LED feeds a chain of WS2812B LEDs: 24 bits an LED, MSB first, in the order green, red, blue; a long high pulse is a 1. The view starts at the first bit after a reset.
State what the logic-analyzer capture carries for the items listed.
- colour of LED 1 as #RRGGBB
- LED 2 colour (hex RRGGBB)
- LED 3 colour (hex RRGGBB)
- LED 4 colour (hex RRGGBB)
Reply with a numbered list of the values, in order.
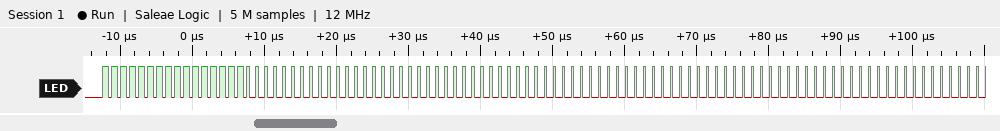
1. #FFFF00
2. #000000
3. #000000
4. #000000
